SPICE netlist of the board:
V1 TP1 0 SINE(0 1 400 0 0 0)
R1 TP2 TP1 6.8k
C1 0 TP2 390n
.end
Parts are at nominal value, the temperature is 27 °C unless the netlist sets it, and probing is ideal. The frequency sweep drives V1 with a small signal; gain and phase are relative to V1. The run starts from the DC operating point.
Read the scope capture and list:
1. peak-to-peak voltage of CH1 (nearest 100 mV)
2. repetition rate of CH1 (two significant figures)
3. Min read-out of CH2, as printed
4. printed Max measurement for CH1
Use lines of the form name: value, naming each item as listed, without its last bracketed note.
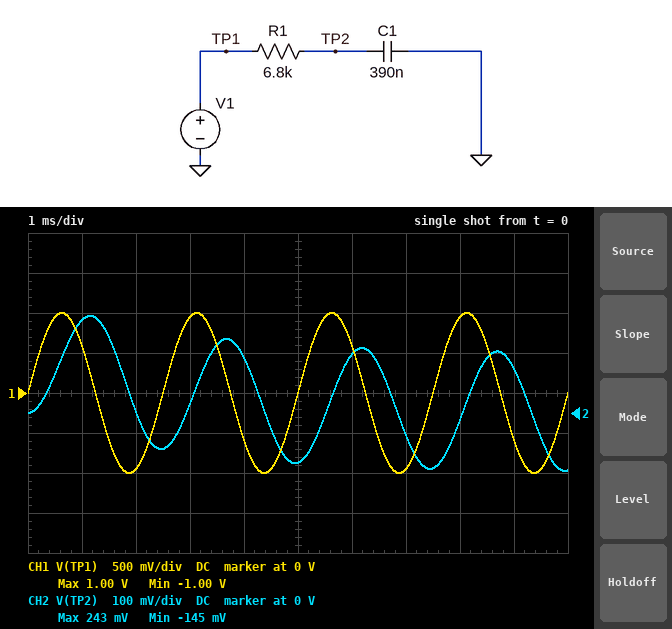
peak-to-peak voltage of CH1: 2.0 V
repetition rate of CH1: 400 Hz
Min read-out of CH2, as printed: -145 mV
printed Max measurement for CH1: 1.00 V
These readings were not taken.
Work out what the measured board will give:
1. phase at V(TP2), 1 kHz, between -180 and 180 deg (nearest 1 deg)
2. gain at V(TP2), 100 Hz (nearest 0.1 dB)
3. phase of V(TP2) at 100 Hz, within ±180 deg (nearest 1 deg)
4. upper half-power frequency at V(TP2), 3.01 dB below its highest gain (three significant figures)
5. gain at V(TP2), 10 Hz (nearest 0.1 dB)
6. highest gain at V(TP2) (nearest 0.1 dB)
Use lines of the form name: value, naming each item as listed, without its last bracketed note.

phase at V(TP2), 1 kHz, between -180 and 180 deg: -87 deg
gain at V(TP2), 100 Hz: -5.8 dB
phase of V(TP2) at 100 Hz, within ±180 deg: -59 deg
upper half-power frequency at V(TP2), 3.01 dB below its highest gain: 60.0 Hz
gain at V(TP2), 10 Hz: -0.1 dB
highest gain at V(TP2): 0 dB
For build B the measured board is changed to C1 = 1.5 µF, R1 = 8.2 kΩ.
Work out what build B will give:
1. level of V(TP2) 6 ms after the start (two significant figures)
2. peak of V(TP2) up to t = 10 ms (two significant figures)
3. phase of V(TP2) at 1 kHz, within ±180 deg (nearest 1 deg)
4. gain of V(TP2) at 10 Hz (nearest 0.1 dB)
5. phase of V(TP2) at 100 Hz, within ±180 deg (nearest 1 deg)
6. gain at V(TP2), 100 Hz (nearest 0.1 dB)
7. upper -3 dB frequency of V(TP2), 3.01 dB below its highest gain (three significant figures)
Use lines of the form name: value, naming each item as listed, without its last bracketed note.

level of V(TP2) 6 ms after the start: 47 mV
peak of V(TP2) up to t = 10 ms: 62 mV
phase of V(TP2) at 1 kHz, within ±180 deg: -89 deg
gain of V(TP2) at 10 Hz: -2.0 dB
phase of V(TP2) at 100 Hz, within ±180 deg: -83 deg
gain at V(TP2), 100 Hz: -17.8 dB
upper -3 dB frequency of V(TP2), 3.01 dB below its highest gain: 12.9 Hz
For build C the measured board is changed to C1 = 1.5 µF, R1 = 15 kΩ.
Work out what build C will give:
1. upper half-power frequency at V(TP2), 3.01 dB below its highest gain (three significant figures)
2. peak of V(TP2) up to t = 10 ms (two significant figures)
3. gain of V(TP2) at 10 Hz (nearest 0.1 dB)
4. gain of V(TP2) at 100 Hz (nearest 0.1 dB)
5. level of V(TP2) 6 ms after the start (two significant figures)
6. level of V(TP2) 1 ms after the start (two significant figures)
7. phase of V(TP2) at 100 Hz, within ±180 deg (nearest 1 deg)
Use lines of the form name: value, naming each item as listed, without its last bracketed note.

upper half-power frequency at V(TP2), 3.01 dB below its highest gain: 7.07 Hz
peak of V(TP2) up to t = 10 ms: 34 mV
gain of V(TP2) at 10 Hz: -4.8 dB
gain of V(TP2) at 100 Hz: -23.0 dB
level of V(TP2) 6 ms after the start: 28 mV
level of V(TP2) 1 ms after the start: 31 mV
phase of V(TP2) at 100 Hz, within ±180 deg: -86 deg
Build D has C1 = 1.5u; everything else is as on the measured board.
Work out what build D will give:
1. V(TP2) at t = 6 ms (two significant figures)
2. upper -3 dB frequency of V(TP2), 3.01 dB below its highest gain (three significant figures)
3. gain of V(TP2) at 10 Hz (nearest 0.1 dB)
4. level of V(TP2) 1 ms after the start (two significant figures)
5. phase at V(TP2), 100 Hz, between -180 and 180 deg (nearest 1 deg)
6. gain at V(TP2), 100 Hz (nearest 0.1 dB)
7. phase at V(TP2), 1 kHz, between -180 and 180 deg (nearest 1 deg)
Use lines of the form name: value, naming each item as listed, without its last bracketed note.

V(TP2) at t = 6 ms: 54 mV
upper -3 dB frequency of V(TP2), 3.01 dB below its highest gain: 15.6 Hz
gain of V(TP2) at 10 Hz: -1.5 dB
level of V(TP2) 1 ms after the start: 68 mV
phase at V(TP2), 100 Hz, between -180 and 180 deg: -81 deg
gain at V(TP2), 100 Hz: -16.2 dB
phase at V(TP2), 1 kHz, between -180 and 180 deg: -89 deg
